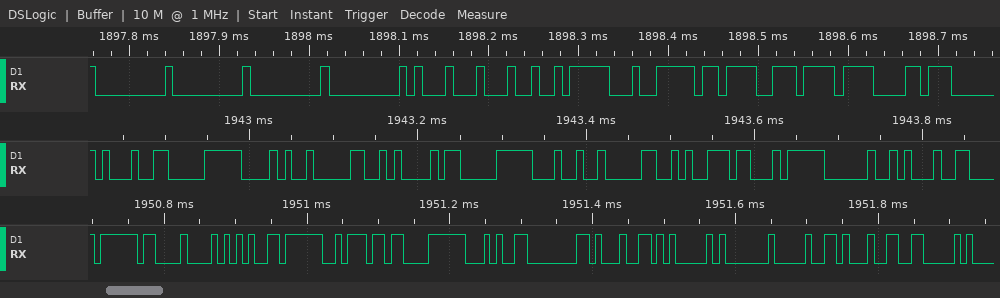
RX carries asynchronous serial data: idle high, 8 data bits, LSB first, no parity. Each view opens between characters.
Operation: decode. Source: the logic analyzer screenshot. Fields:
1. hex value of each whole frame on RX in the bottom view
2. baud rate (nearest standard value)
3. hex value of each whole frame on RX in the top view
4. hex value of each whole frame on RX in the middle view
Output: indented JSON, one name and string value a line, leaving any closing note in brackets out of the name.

{
  "hex value of each whole frame on RX in the bottom view": "BF, 08, 95, 3F, B7, F8, 94, 80, 91, 05, 01, 90, 91, 06",
  "baud rate": "115200 baud",
  "hex value of each whole frame on RX in the top view": "00, 00, 00, 00, 11, 24, 1F, BE, CF, EF, D8",
  "hex value of each whole frame on RX in the middle view": "91, F0, 28, 30, A1, F0, 24, 30, B9, F4, 20, 91"
}
